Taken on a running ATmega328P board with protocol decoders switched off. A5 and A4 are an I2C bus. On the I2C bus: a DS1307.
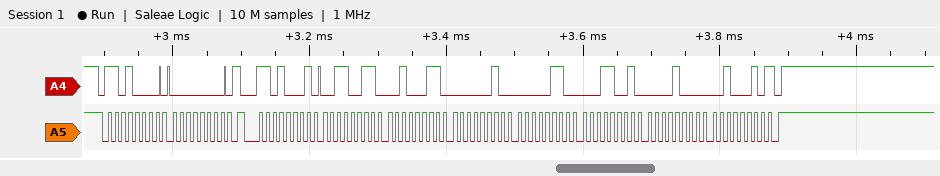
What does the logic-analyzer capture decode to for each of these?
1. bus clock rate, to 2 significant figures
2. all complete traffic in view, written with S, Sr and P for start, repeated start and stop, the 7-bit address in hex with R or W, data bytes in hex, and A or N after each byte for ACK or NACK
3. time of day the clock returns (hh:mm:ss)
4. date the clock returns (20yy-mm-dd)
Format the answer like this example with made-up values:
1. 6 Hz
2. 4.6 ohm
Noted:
1. 100 kHz
2. S 68W A 00 A Sr 68R A 33 A 23 A 02 A 06 A 19 A 08 A 22 N P
3. 02:23:33
4. 2022-08-19
